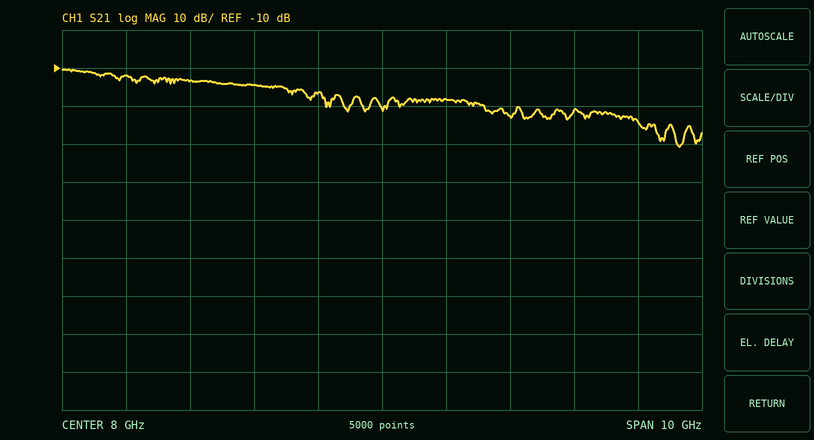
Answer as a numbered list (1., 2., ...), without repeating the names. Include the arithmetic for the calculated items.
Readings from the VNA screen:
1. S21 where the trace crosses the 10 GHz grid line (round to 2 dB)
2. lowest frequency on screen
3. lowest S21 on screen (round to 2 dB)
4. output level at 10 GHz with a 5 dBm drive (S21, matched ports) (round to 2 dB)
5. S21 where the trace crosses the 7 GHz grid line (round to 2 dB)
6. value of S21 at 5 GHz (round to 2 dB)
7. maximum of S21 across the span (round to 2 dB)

1. -22 dB
2. 3 GHz
3. -30 dB
4. 5 dBm + (-22 dB) = -18 dBm
5. -16 dB
6. -14 dB
7. -10 dB
